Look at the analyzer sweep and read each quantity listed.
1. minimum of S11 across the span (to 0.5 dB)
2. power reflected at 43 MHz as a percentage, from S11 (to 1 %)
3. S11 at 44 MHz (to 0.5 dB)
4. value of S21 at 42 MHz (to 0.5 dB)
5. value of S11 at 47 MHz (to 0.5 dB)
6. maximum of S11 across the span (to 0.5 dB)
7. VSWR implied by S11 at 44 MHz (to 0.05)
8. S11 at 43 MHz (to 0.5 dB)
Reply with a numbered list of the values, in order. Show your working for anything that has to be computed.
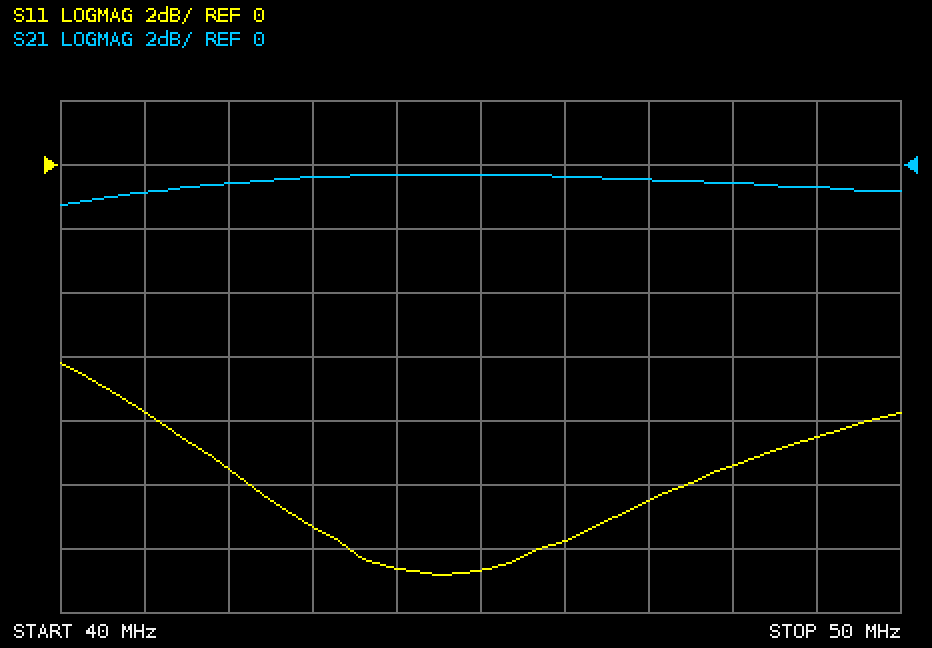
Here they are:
1. -13.0 dB
2. 10^(-11.5/10) ≈ 7 %
3. -12.5 dB
4. -0.5 dB
5. -10.5 dB
6. -6.0 dB
7. |Γ| = 10^(-12.5/20) = 0.2371; VSWR = (1 + 0.2371)/(1 − 0.2371) ≈ 1.62, so 1.60 to the nearest 0.05
8. -11.5 dB
